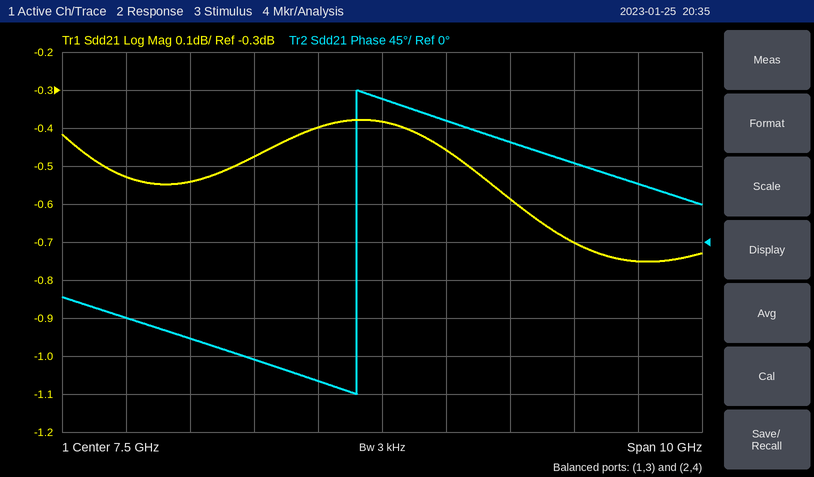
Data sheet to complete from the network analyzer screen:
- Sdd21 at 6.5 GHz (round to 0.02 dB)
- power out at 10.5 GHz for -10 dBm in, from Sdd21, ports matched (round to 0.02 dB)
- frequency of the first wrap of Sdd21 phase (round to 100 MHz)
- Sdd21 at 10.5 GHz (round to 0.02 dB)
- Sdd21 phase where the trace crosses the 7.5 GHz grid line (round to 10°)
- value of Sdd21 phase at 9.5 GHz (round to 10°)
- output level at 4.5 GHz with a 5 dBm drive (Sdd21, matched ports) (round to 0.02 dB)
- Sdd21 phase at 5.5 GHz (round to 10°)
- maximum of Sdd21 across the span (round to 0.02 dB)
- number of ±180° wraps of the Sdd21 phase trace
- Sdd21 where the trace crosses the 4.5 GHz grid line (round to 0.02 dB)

-0.40 dB
-10.70 dBm
7.1 GHz
-0.70 dB
170°
120°
4.46 dBm
-140°
-0.38 dB
1
-0.54 dB
